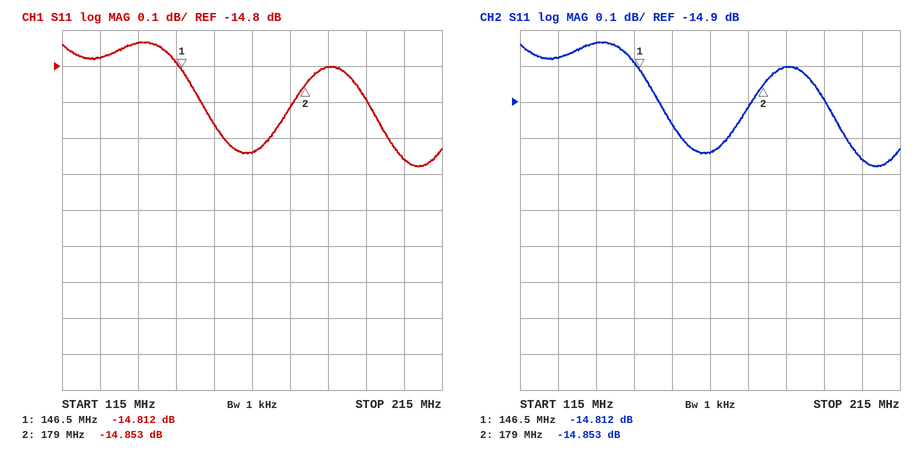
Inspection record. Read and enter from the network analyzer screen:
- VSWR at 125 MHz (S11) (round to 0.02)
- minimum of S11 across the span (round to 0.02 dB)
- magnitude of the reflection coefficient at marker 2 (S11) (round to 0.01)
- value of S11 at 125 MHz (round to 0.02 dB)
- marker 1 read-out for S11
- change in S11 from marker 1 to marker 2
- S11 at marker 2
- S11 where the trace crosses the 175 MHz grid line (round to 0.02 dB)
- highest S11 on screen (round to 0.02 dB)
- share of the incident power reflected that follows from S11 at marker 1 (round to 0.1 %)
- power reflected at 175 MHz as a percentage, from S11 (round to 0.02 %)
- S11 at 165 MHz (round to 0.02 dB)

1.44
-15.08 dB
0.18
-14.78 dB
-14.812 dB
-0.041 dB
-14.853 dB
-14.92 dB
-14.74 dB
3.3 %
3.22 %
-15.04 dB
